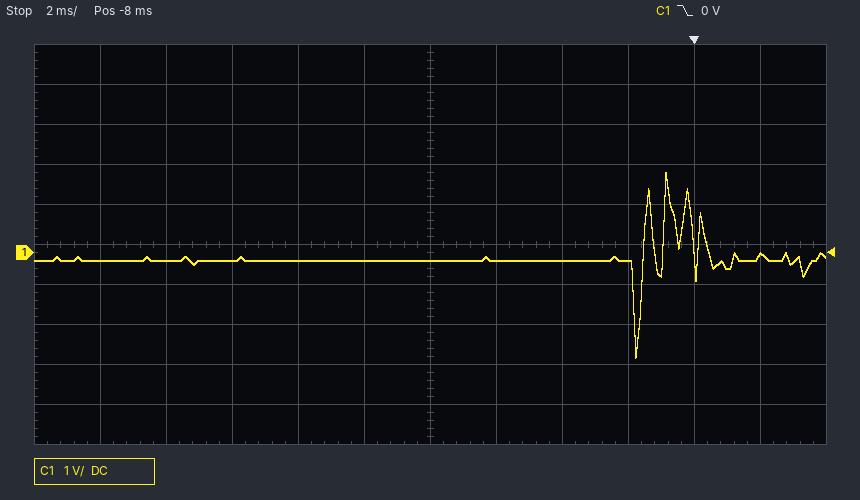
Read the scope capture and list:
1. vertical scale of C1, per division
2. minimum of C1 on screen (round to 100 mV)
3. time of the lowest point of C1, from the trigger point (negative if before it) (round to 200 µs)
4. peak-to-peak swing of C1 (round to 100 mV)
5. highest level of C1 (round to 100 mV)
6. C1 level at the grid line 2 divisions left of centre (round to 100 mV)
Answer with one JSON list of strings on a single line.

["1 V", "-2.6 V", "-1.8 ms", "4.6 V", "2.0 V", "-200 mV"]
